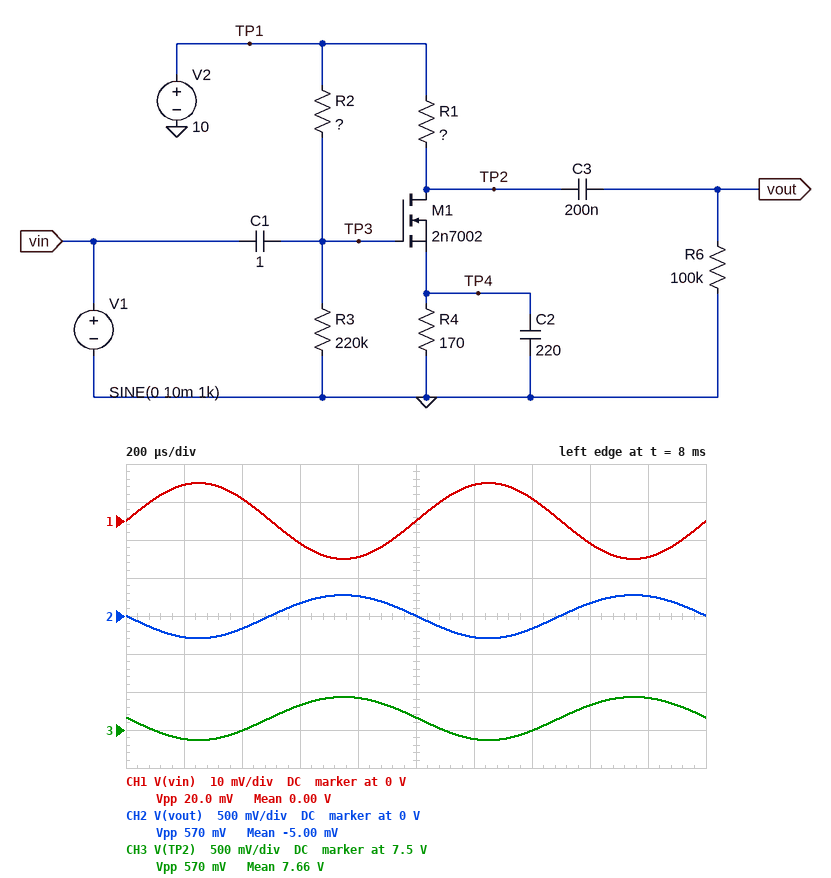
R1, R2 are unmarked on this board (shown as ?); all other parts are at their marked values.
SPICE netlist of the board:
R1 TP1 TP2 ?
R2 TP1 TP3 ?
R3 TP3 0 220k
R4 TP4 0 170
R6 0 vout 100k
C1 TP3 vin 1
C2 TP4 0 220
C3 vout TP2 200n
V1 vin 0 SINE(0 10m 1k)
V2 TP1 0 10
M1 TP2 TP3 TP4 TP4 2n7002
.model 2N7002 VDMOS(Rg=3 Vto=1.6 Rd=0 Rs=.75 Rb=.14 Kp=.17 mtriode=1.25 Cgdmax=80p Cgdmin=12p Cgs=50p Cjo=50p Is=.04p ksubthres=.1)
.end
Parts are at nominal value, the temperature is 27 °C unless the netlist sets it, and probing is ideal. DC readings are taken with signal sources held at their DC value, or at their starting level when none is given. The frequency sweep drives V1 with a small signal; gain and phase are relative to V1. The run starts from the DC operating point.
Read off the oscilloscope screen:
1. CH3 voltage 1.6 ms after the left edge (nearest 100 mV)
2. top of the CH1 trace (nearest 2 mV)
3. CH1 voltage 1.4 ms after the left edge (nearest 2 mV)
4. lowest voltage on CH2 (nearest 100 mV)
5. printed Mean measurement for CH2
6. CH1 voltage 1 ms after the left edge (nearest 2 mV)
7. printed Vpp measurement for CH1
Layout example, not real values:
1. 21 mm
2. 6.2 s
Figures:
1. 7.8 V
2. 10 mV
3. 6 mV
4. -300 mV
5. -5.00 mV
6. 0 V
7. 20.0 mV
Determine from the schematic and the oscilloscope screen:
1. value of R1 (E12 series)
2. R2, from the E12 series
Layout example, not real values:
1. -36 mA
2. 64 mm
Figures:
1. 2.7 kΩ
2. 1 MΩ
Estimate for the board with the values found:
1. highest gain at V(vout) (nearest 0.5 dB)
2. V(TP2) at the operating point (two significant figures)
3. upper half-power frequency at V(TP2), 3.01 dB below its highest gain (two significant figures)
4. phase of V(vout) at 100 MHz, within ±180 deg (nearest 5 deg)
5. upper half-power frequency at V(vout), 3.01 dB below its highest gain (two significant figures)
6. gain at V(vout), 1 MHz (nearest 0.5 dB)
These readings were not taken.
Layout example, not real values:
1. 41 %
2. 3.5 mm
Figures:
1. 29.0 dB
2. 7.7 V
3. 1.8 MHz
4. 40 deg
5. 1.9 MHz
6. 28.0 dB
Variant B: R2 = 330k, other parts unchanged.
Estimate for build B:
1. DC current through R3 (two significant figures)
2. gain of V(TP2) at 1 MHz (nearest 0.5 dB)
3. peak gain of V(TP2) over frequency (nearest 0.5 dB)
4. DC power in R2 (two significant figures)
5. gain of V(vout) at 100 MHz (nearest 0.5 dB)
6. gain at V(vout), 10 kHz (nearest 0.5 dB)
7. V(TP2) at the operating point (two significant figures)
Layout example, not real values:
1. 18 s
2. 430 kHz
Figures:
1. 18 µA
2. -45.5 dB
3. -9.0 dB
4. 110 µW
5. -15.0 dB
6. -46.0 dB
7. 600 mV
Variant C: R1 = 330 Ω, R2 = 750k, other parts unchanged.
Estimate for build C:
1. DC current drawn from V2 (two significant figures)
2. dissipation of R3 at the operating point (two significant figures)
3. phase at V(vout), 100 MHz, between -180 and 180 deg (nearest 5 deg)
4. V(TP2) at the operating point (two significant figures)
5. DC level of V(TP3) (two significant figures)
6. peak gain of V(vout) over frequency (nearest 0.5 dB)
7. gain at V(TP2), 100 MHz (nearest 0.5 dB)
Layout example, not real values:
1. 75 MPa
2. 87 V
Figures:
1. 2.9 mA
2. 23 µW
3. 70 deg
4. 9.0 V
5. 2.3 V
6. 18.5 dB
7. 3.0 dB
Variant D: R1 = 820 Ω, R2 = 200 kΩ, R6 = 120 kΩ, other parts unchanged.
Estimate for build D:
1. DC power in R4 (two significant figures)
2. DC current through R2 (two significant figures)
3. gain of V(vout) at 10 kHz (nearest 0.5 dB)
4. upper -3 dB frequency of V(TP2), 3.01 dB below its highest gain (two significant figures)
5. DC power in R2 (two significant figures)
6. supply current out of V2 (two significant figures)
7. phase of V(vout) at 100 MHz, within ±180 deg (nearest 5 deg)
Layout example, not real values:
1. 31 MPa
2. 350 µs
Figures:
1. 17 mW
2. 24 µA
3. -37.5 dB
4. 1.6 GHz
5. 110 µW
6. 10 mA
7. 65 deg
